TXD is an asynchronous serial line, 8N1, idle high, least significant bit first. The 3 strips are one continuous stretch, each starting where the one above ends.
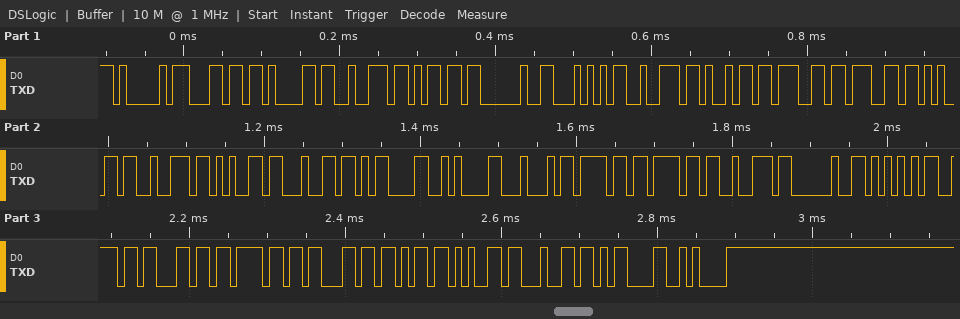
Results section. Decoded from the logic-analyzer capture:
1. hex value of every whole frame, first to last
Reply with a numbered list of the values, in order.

1. 0x41 0x6C 0x61 0x72 0x6D 0x20 0x54 0x72 0x69 0x67 0x67 0x65 0x72 0x65 0x64 0x0D 0x0A 0x44 0x6F 0x6F 0x72 0x20 0x55 0x6E 0x6C 0x6F 0x63 0x6B 0x65 0x64 0x0D 0x0A
